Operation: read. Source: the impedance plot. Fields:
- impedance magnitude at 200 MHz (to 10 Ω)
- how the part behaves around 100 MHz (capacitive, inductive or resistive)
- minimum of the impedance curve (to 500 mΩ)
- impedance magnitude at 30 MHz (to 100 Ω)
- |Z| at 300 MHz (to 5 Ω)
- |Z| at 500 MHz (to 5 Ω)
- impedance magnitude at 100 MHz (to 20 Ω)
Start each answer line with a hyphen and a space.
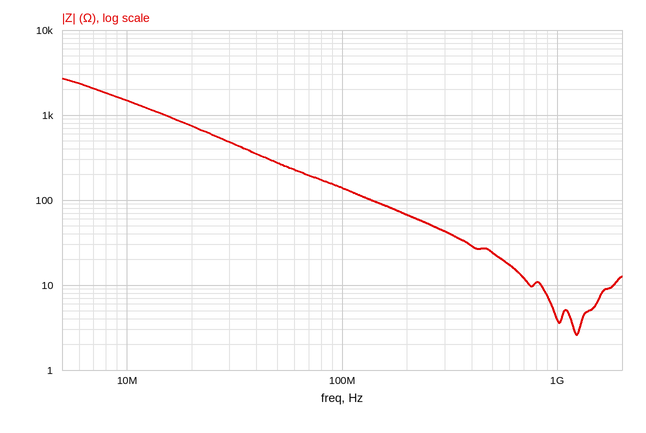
- 70 Ω
- capacitive
- 2.5 Ω
- 500 Ω
- 45 Ω
- 25 Ω
- 140 Ω
